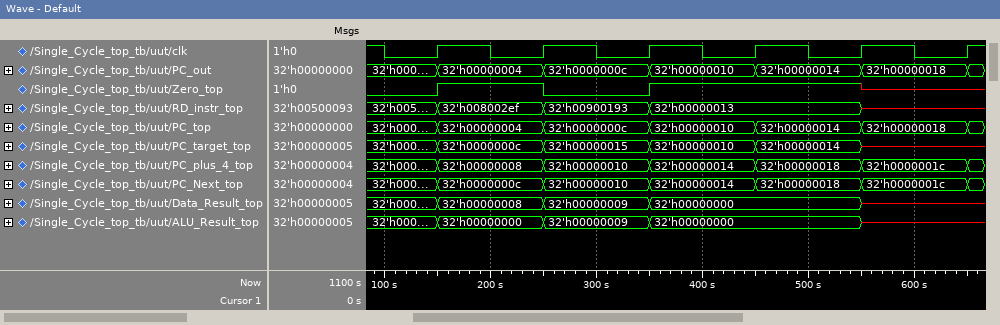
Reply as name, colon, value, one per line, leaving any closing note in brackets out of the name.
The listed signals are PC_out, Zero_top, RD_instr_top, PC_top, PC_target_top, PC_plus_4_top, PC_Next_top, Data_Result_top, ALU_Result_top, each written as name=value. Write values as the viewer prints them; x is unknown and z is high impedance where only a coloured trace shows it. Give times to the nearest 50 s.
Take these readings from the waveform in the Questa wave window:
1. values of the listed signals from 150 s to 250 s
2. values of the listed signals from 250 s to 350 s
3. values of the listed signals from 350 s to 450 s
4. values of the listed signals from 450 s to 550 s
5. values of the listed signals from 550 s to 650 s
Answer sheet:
values of the listed signals from 150 s to 250 s: PC_out=32'h00000004, Zero_top=1, RD_instr_top=32'h008002ef, PC_top=32'h00000004, PC_target_top=32'h0000000c, PC_plus_4_top=32'h00000008, PC_Next_top=32'h0000000c, Data_Result_top=32'h00000008, ALU_Result_top=32'h00000000
values of the listed signals from 250 s to 350 s: PC_out=32'h0000000c, Zero_top=0, RD_instr_top=32'h00900193, PC_top=32'h0000000c, PC_target_top=32'h00000015, PC_plus_4_top=32'h00000010, PC_Next_top=32'h00000010, Data_Result_top=32'h00000009, ALU_Result_top=32'h00000009
values of the listed signals from 350 s to 450 s: PC_out=32'h00000010, Zero_top=1, RD_instr_top=32'h00000013, PC_top=32'h00000010, PC_target_top=32'h00000010, PC_plus_4_top=32'h00000014, PC_Next_top=32'h00000014, Data_Result_top=32'h00000000, ALU_Result_top=32'h00000000
values of the listed signals from 450 s to 550 s: PC_out=32'h00000014, Zero_top=1, RD_instr_top=32'h00000013, PC_top=32'h00000014, PC_target_top=32'h00000014, PC_plus_4_top=32'h00000018, PC_Next_top=32'h00000018, Data_Result_top=32'h00000000, ALU_Result_top=32'h00000000
values of the listed signals from 550 s to 650 s: PC_out=32'h00000018, Zero_top=x, RD_instr_top=x, PC_top=32'h00000018, PC_target_top=x, PC_plus_4_top=32'h0000001c, PC_Next_top=32'h0000001c, Data_Result_top=x, ALU_Result_top=x
